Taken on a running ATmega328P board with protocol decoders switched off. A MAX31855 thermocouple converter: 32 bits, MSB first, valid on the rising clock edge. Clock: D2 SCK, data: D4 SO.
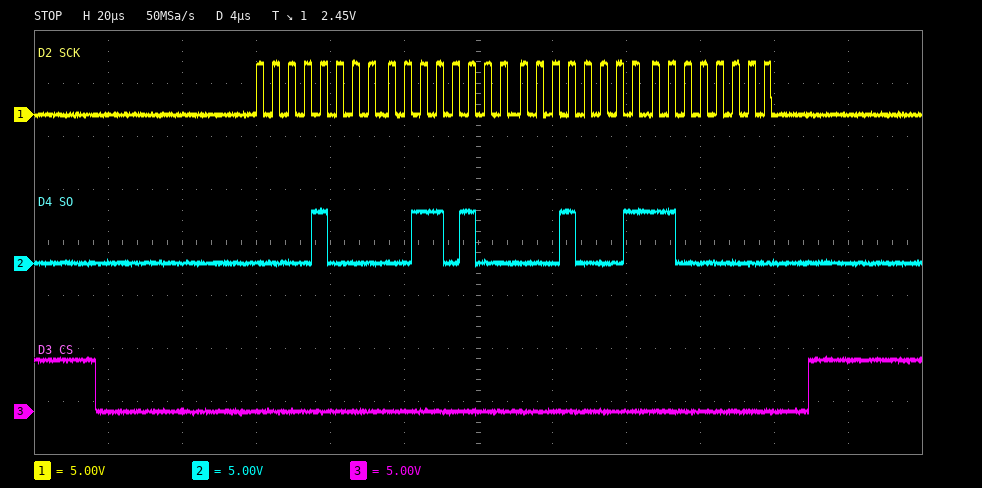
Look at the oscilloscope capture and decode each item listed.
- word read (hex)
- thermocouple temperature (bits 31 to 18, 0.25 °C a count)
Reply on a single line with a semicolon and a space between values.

0x083411C0; 131.25 °C
